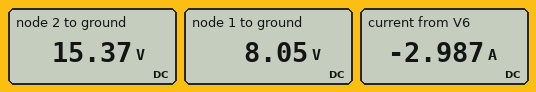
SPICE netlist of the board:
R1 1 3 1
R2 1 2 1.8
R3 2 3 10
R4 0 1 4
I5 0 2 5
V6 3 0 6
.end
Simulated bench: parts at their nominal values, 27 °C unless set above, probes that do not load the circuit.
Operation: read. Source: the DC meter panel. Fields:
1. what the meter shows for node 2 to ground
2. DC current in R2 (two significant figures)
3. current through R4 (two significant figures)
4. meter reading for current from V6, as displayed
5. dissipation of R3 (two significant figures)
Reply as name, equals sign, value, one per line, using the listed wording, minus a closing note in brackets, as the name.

what the meter shows for node 2 to ground = 15.37 V
DC current in R2 = 4.1 A
current through R4 = 2.0 A
meter reading for current from V6, as displayed = -2.987 A
dissipation of R3 = 8.8 W
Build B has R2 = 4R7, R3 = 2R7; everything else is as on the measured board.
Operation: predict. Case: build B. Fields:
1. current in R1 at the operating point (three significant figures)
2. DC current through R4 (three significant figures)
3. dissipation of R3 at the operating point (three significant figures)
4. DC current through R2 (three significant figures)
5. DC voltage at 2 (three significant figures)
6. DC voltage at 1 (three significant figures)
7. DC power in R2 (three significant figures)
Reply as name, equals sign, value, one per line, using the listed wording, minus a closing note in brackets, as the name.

current in R1 at the operating point = 234 mA
DC current through R4 = 1.56 A
dissipation of R3 at the operating point = 27.8 W
DC current through R2 = 1.79 A
DC voltage at 2 = 14.7 V
DC voltage at 1 = 6.23 V
DC power in R2 = 15.1 W
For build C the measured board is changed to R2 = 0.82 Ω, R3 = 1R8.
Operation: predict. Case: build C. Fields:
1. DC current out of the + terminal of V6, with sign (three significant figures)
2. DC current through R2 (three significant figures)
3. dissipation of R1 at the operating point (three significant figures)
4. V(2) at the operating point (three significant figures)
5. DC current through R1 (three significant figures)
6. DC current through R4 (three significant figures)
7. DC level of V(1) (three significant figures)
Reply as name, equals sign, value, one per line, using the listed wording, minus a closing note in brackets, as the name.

DC current out of the + terminal of V6, with sign = -3.20 A
DC current through R2 = 2.98 A
dissipation of R1 at the operating point = 1.41 W
V(2) at the operating point = 9.63 V
DC current through R1 = 1.19 A
DC current through R4 = 1.80 A
DC level of V(1) = 7.19 V
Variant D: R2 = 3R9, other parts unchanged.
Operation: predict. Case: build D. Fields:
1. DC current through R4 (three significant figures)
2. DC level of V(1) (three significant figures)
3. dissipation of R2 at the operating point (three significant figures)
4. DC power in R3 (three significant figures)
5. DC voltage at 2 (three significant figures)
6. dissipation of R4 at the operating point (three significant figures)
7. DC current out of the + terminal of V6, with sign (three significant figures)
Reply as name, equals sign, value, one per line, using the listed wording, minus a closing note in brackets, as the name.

DC current through R4 = 1.90 A
DC level of V(1) = 7.59 V
dissipation of R2 at the operating point = 47.3 W
DC power in R3 = 23.0 W
DC voltage at 2 = 21.2 V
dissipation of R4 at the operating point = 14.4 W
DC current out of the + terminal of V6, with sign = -3.10 A
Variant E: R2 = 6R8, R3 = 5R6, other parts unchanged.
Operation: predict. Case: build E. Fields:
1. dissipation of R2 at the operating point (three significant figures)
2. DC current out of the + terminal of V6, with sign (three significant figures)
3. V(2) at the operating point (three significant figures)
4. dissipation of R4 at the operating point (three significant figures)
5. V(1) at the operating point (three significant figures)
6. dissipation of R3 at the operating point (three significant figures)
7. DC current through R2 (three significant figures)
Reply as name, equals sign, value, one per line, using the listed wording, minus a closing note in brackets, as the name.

dissipation of R2 at the operating point = 33.3 W
DC current out of the + terminal of V6, with sign = -3.36 A
V(2) at the operating point = 21.6 V
dissipation of R4 at the operating point = 10.8 W
V(1) at the operating point = 6.57 V
dissipation of R3 at the operating point = 43.5 W
DC current through R2 = 2.21 A
